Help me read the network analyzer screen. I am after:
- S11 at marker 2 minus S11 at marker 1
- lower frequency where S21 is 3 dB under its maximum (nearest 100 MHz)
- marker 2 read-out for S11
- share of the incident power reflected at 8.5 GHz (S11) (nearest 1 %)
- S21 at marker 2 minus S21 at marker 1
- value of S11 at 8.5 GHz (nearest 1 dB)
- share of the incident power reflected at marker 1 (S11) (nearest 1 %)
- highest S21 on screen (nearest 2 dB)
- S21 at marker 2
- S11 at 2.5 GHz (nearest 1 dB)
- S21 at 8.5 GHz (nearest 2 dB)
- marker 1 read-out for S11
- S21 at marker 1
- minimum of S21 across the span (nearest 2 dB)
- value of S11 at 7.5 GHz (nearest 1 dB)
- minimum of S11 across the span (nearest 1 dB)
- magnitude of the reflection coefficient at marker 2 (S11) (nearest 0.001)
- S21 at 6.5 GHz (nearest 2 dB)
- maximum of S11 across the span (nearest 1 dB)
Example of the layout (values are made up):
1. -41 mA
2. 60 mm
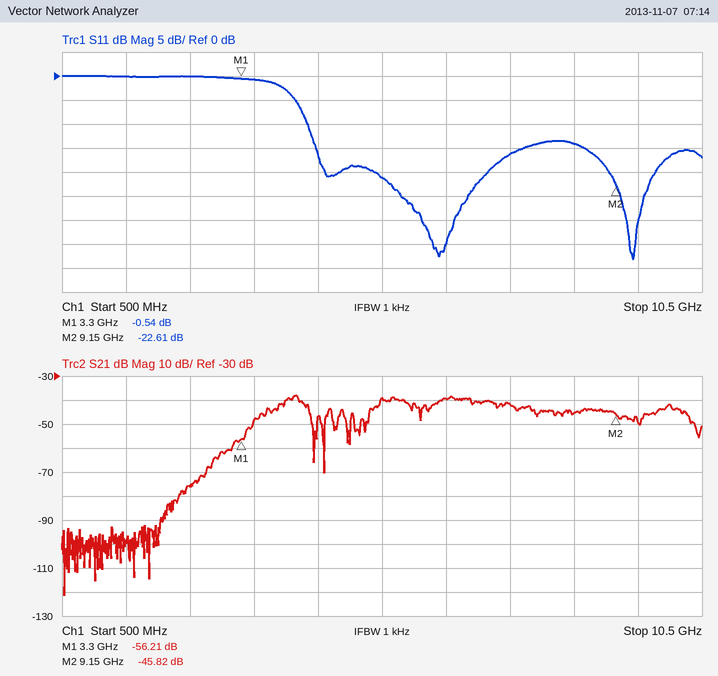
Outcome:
1. -22.07 dB
2. 4.0 GHz
3. -22.61 dB
4. 4 %
5. 10.39 dB
6. -14 dB
7. 88 %
8. -38 dB
9. -45.82 dB
10. 0 dB
11. -46 dB
12. -0.54 dB
13. -56.21 dB
14. -122 dB
15. -16 dB
16. -38 dB
17. 0.074
18. -40 dB
19. 0 dB
